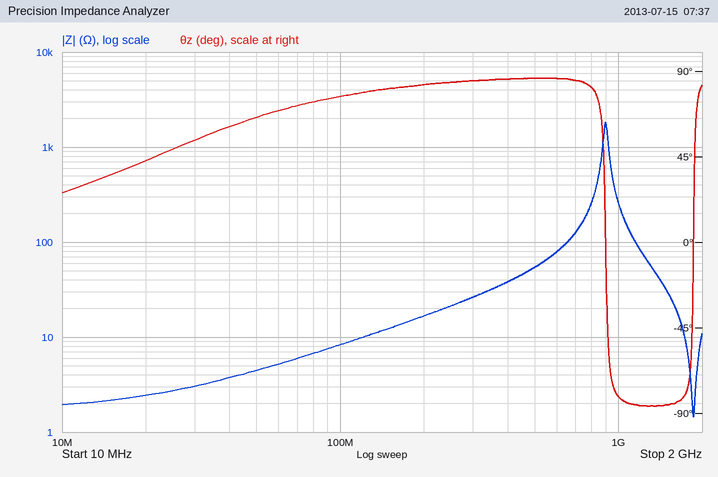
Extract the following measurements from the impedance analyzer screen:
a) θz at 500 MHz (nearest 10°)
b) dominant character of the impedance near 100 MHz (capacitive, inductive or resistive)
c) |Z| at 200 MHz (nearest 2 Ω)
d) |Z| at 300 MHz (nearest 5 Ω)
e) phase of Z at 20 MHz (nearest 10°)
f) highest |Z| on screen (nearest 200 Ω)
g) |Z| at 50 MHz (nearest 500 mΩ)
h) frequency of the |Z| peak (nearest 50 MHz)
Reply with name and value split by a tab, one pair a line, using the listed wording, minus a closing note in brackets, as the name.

θz at 500 MHz	90°
dominant character of the impedance near 100 MHz	inductive
|Z| at 200 MHz	16 Ω
|Z| at 300 MHz	25 Ω
phase of Z at 20 MHz	40°
highest |Z| on screen	1.8 kΩ
|Z| at 50 MHz	4.5 Ω
frequency of the |Z| peak	900 MHz
